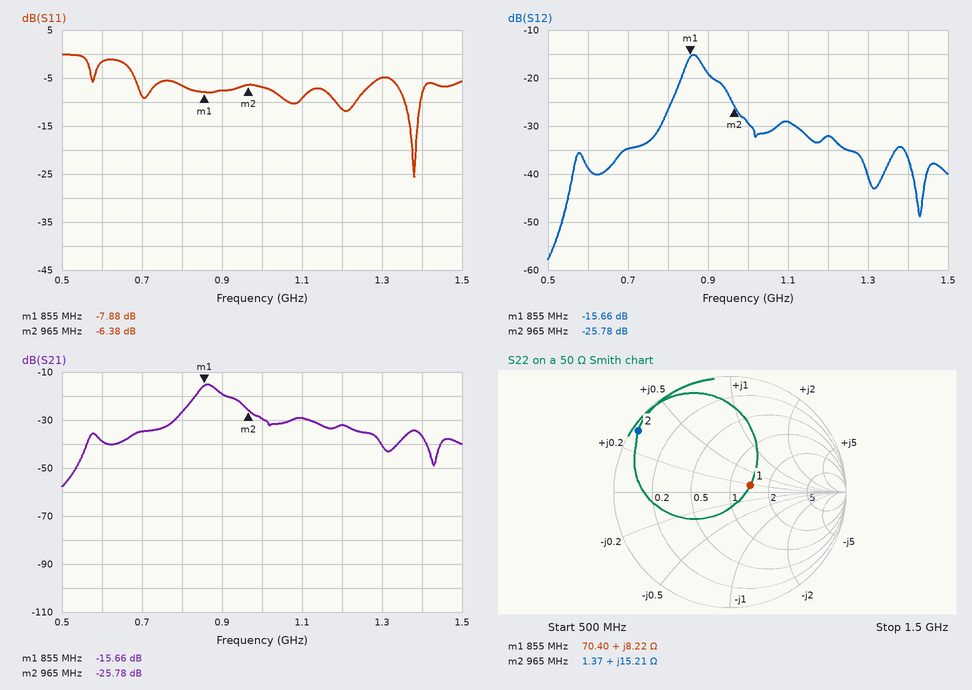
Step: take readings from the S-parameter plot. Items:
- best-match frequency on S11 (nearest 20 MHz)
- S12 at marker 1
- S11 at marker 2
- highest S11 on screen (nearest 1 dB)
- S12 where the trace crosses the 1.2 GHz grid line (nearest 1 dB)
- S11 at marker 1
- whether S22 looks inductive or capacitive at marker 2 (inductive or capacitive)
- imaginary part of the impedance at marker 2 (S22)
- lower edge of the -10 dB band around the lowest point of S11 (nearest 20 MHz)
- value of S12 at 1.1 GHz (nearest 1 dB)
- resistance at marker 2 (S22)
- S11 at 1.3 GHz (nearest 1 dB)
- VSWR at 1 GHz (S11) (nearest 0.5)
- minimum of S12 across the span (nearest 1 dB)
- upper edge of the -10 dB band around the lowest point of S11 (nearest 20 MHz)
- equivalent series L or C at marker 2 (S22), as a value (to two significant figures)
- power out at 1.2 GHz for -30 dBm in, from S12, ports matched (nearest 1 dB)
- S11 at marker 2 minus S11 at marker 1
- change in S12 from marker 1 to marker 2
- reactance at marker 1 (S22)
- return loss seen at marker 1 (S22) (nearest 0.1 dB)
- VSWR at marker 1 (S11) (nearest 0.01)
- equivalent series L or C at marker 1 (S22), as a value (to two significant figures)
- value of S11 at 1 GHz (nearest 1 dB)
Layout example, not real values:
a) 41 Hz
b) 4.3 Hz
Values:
a) 1.38 GHz
b) -15.66 dB
c) -6.38 dB
d) 0 dB
e) -32 dB
f) -7.88 dB
g) inductive
h) +15.21 Ω
i) 1.36 GHz
j) -29 dB
k) 1.37 Ω
l) -5 dB
m) 2.5
n) -58 dB
o) 1.40 GHz
p) 2.5 nH
q) -62 dBm
r) 1.50 dB
s) -10.12 dB
t) +8.22 Ω
u) 14.8 dB
v) 2.35
w) 1.5 nH
x) -7 dB
